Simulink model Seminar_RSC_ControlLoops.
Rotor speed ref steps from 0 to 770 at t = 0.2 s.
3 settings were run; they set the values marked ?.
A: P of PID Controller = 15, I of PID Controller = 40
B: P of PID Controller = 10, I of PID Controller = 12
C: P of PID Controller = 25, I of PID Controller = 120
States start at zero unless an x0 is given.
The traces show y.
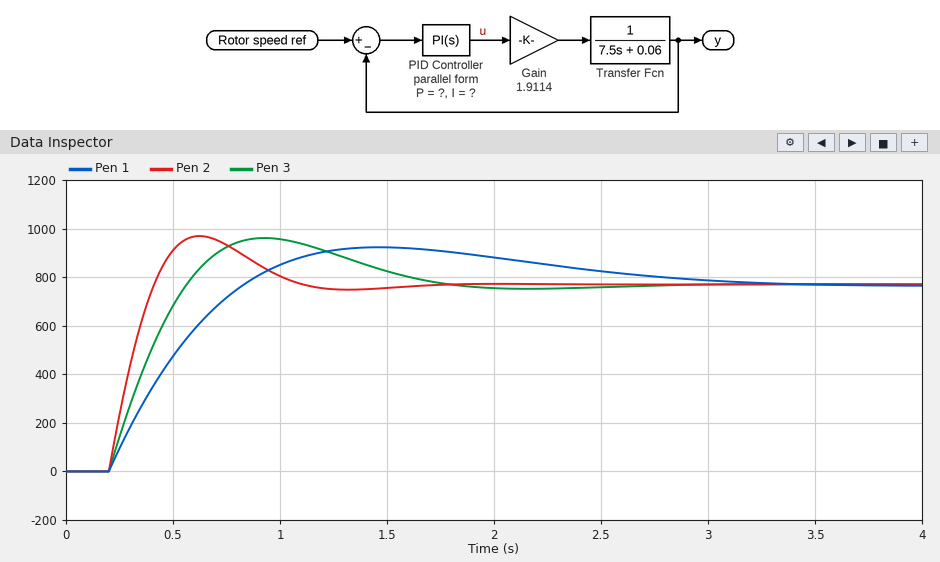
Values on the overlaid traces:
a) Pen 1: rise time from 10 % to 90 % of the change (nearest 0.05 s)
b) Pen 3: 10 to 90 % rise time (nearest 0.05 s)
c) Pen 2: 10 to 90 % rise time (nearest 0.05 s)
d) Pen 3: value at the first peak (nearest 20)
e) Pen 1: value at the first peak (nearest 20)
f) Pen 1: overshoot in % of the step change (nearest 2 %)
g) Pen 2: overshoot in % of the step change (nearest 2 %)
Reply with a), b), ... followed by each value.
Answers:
a) 0.50 s
b) 0.30 s
c) 0.15 s
d) 960
e) 920
f) 20 %
g) 26 %
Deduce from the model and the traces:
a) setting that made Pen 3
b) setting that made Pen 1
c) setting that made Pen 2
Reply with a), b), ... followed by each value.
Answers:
a) A
b) B
c) C
